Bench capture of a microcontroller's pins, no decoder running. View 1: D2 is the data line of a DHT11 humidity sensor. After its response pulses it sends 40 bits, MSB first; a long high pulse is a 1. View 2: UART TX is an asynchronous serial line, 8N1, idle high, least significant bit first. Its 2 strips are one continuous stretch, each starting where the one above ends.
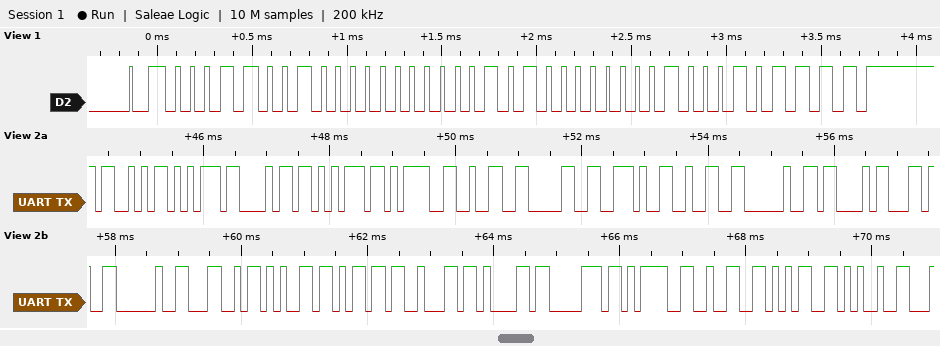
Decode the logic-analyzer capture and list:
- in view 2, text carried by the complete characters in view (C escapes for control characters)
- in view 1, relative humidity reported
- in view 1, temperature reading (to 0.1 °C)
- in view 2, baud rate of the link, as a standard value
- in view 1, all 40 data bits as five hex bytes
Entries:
"Suhu=20.2 C, Lembap=25%"
25 %
20.2 °C
9600 baud
19 00 14 02 2F
